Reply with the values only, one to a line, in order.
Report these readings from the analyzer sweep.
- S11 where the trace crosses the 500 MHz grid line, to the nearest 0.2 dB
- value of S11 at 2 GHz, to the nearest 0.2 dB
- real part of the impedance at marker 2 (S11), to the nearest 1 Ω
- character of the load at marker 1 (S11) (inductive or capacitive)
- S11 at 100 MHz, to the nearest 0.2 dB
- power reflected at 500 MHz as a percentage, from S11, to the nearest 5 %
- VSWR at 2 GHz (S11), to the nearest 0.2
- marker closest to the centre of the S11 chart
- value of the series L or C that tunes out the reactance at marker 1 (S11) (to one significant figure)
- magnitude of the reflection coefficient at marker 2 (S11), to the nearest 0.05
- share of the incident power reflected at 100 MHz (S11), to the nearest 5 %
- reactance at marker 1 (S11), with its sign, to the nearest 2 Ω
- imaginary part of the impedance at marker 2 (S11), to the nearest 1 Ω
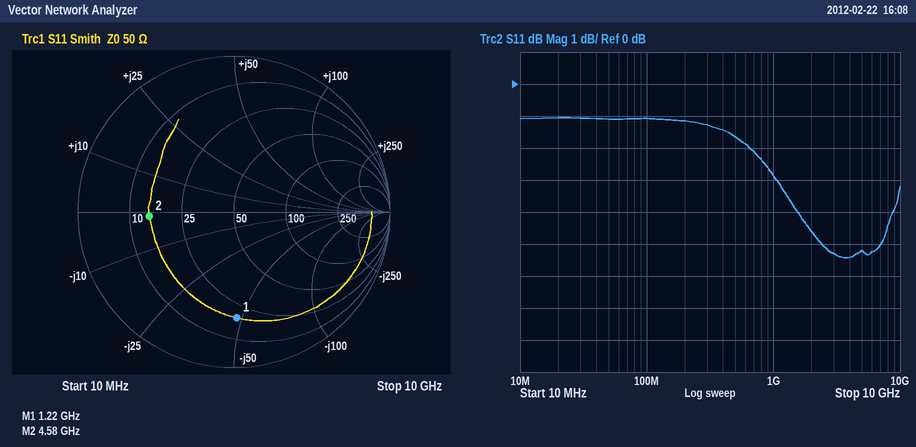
-1.6 dB
-4.6 dB
15 Ω
capacitive
-1.0 dB
70 %
3.8
marker 2
6 nH
0.55
80 %
-48 Ω
-1 Ω
